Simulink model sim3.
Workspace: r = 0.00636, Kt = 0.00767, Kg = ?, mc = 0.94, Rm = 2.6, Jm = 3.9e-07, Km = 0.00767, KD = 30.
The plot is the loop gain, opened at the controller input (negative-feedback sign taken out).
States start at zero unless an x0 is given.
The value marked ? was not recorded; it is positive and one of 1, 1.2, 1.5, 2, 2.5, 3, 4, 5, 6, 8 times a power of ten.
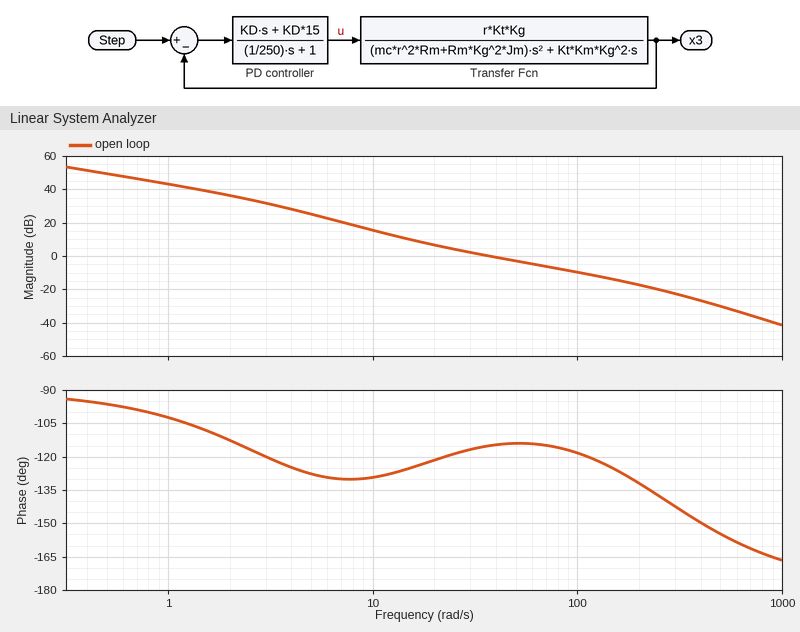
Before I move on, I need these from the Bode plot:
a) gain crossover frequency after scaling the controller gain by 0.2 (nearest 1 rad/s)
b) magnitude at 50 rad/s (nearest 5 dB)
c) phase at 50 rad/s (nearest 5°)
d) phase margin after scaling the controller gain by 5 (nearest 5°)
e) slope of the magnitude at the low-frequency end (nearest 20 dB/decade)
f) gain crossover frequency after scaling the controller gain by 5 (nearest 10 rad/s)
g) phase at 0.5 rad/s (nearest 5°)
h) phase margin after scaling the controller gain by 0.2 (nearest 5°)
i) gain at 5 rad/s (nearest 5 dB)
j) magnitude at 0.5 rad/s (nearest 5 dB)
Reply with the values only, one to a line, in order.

11 rad/s
-5 dB
-115°
55°
-20 dB/decade
150 rad/s
-95°
50°
25 dB
50 dB
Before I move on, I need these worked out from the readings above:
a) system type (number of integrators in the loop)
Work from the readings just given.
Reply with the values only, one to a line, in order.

1
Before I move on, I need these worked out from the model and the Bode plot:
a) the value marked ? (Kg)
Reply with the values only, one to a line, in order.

2.5
